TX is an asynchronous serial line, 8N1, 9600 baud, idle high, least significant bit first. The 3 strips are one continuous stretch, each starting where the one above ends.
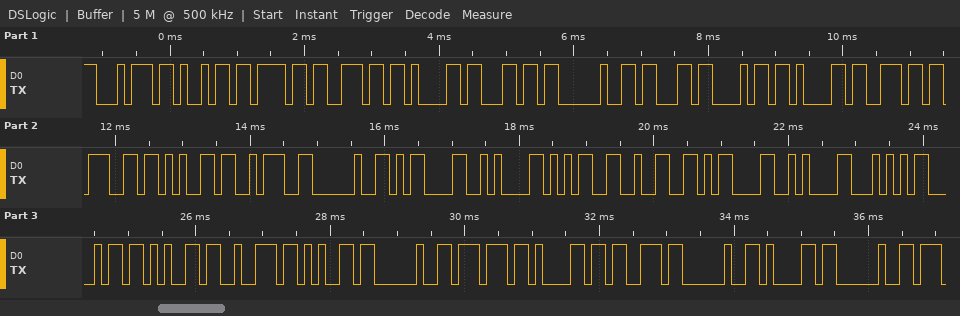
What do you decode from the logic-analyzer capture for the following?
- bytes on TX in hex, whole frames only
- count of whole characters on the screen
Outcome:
74 69 6F 6E 61 6C 20 63 68 61 6E 67 65 3A 20 0D 0A 35 32 0D 0A 54 68 65 72 65 20 77 61 73 20 61 20
33
